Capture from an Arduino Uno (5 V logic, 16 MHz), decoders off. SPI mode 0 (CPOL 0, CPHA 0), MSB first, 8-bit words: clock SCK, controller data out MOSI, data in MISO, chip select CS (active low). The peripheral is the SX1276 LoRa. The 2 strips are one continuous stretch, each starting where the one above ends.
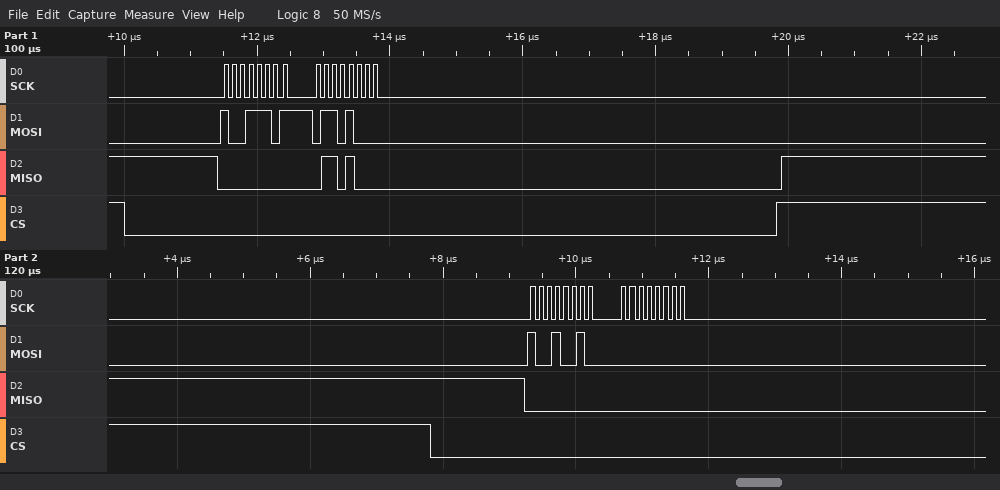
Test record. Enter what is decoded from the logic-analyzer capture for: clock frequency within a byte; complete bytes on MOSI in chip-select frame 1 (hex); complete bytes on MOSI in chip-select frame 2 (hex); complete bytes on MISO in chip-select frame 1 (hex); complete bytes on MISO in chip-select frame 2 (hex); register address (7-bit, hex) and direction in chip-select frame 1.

8 MHz
9D 68
92 00
00 68
00 00
0x1D write
